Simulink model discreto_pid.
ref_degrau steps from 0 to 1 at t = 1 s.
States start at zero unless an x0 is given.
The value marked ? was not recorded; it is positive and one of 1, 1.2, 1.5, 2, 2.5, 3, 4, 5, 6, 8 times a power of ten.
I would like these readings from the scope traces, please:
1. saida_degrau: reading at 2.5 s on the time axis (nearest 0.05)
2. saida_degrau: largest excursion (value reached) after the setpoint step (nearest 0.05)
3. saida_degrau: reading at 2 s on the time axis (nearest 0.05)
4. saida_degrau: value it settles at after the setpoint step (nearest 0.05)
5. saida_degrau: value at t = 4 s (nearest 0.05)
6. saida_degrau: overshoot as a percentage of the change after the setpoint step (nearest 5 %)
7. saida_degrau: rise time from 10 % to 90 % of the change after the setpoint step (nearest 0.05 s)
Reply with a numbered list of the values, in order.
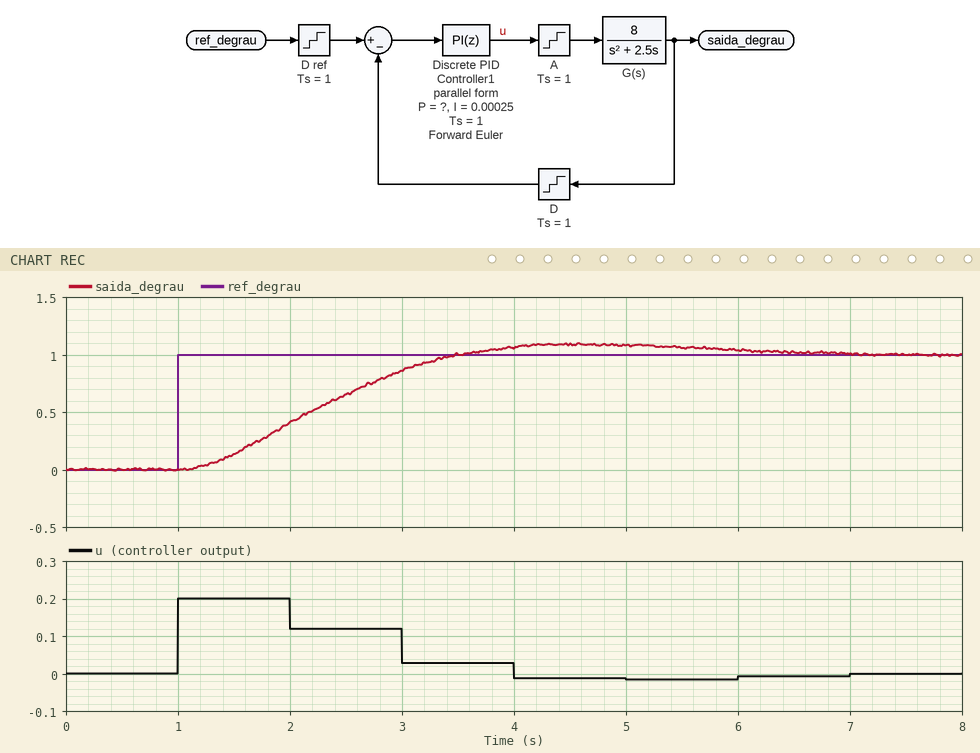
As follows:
1. 0.65
2. 1.10
3. 0.40
4. 1.00
5. 1.05
6. 10 %
7. 1.70 s
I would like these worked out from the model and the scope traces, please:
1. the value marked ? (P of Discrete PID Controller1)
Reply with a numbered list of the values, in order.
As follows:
1. 0.2
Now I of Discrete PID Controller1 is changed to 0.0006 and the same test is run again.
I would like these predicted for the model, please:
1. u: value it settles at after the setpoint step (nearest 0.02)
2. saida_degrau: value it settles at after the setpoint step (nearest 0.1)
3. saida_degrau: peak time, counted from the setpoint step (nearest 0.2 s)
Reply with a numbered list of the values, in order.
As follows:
1. 0.00
2. 1.0
3. 3.6 s
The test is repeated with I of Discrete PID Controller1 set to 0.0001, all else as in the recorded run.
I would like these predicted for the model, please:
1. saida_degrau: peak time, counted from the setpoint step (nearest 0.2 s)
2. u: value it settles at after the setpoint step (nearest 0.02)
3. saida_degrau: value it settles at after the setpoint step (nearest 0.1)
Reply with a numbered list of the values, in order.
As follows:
1. 3.6 s
2. 0.00
3. 1.0
